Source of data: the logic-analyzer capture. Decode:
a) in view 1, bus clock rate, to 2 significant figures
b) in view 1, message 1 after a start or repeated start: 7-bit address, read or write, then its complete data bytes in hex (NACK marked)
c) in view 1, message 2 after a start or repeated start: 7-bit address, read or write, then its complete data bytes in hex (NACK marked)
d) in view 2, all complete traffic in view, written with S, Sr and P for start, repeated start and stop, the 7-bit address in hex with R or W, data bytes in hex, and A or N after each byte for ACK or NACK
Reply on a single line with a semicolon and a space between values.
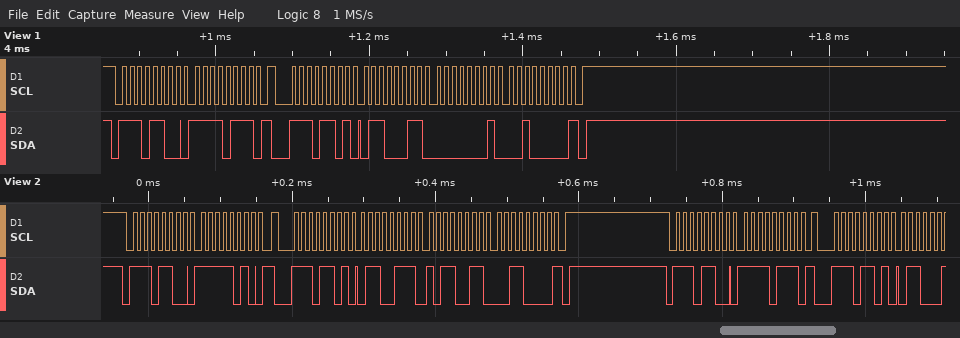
100 kHz; 0x76 write: F7; 0x76 read: 63 01 20 NACK; S 76W A FA A Sr 76R A 67 A B3 A 30 N P S 76W A F7 A Sr 76R A
